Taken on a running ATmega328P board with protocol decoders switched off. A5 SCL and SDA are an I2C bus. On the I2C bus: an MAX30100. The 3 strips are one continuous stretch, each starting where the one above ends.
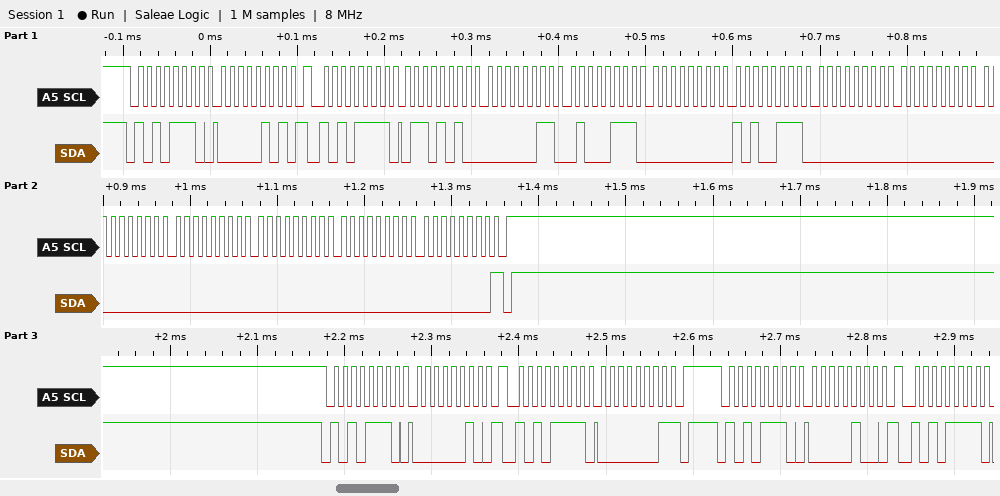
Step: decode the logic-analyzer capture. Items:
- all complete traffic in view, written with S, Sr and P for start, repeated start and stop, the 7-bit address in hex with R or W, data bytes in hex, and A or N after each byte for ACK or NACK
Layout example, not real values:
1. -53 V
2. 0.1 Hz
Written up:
1. S 57W A 05 A Sr 57R A 6A A 03 A 47 A 00 A A7 A 00 A 00 A 00 A 00 A 00 A 00 A 00 N P S 57W A 02 A Sr 57R A 01 N P S 57W A 04 A Sr 57R A
